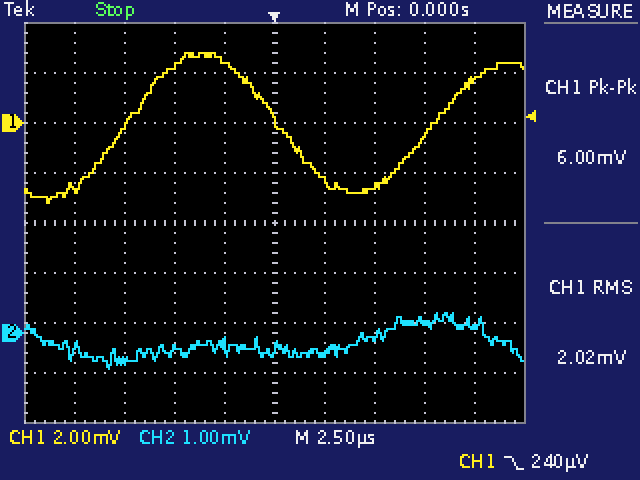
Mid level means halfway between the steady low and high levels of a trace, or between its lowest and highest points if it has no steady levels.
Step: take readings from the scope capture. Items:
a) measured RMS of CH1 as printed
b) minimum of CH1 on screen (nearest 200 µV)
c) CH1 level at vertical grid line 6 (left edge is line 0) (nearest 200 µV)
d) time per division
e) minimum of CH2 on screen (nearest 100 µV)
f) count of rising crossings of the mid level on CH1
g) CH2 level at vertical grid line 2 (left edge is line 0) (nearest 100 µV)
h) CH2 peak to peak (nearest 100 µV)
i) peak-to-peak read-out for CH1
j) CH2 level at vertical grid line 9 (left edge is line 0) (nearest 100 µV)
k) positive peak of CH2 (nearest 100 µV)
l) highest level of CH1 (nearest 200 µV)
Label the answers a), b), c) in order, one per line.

a) 2.02 mV
b) -3.2 mV
c) -2.4 mV
d) 2.5 µs
e) -700 µV
f) 2
g) -600 µV
h) 1.1 mV
i) 6.00 mV
j) 100 µV
k) 400 µV
l) 2.8 mV
